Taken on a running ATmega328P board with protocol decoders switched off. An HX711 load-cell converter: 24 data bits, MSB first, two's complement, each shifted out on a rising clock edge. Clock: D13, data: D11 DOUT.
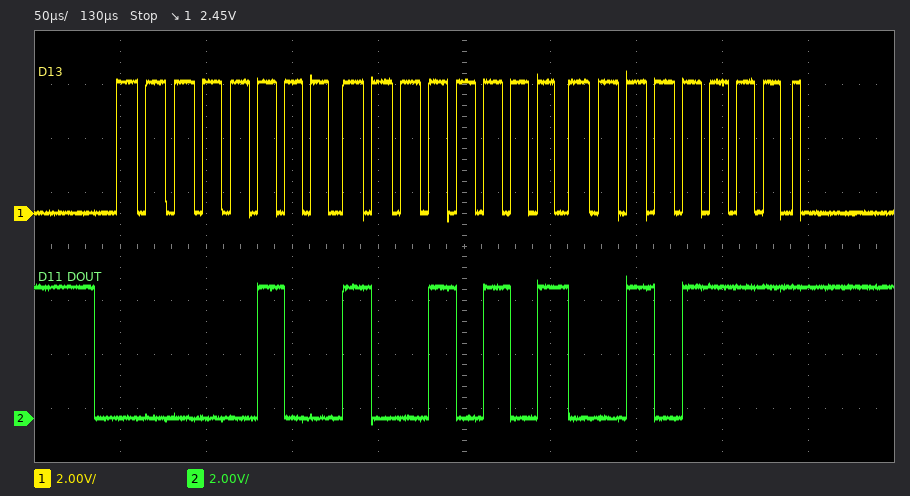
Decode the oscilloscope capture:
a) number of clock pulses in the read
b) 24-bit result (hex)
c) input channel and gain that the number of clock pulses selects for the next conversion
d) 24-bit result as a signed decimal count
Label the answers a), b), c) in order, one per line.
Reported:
a) 25
b) 0x04952F
c) channel A, gain 128
d) 300335
